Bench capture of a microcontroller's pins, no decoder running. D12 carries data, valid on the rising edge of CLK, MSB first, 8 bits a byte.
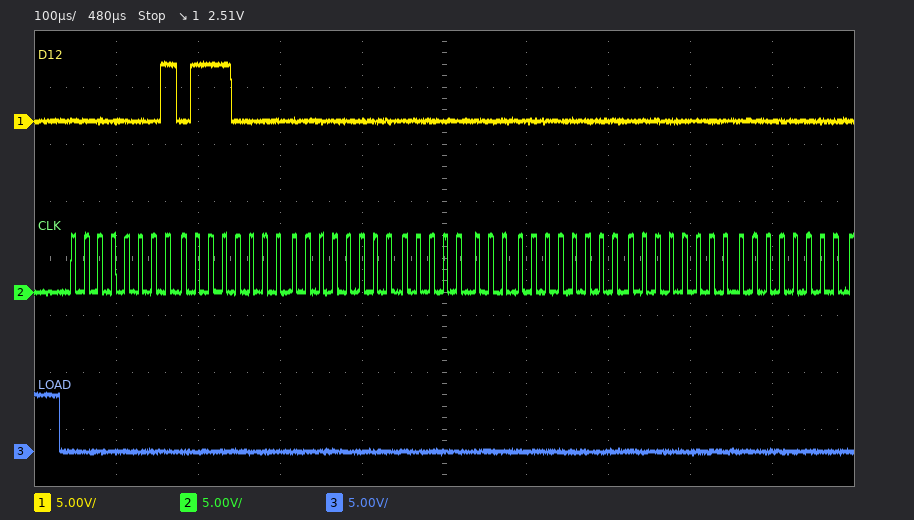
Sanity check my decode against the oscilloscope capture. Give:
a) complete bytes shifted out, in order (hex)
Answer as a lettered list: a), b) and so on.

a) 01 70 00 00 00 00 00
